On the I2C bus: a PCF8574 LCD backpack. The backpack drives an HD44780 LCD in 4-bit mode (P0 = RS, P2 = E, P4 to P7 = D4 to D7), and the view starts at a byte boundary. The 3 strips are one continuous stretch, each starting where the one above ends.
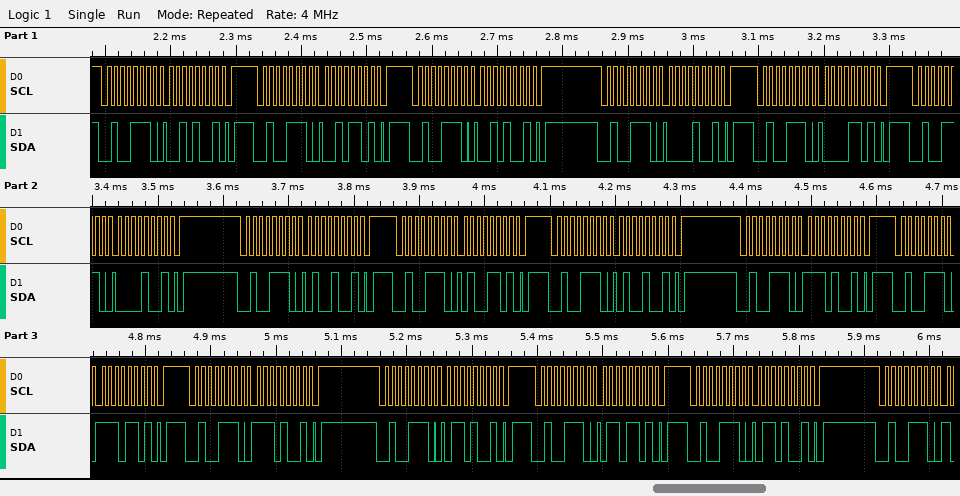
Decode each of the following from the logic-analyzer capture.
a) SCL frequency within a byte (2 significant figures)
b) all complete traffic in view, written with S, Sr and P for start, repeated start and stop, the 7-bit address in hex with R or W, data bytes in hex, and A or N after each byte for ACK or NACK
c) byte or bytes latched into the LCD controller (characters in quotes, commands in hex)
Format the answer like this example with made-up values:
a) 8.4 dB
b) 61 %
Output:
a) 100 kHz
b) S 27W A 29 A P S 27W A 2D A P S 27W A 29 A P S 27W A 09 A P S 27W A 0D A P S 27W A 09 A P S 27W A 49 A P S 27W A 4D A P S 27W A 49 A P S 27W A E9 A P S 27W A ED A P S 27W A E9 A P S 27W A 69 A P S 27W A 6D A P S 27W A 69 A P S 27W A
c) ' ' 'N'
